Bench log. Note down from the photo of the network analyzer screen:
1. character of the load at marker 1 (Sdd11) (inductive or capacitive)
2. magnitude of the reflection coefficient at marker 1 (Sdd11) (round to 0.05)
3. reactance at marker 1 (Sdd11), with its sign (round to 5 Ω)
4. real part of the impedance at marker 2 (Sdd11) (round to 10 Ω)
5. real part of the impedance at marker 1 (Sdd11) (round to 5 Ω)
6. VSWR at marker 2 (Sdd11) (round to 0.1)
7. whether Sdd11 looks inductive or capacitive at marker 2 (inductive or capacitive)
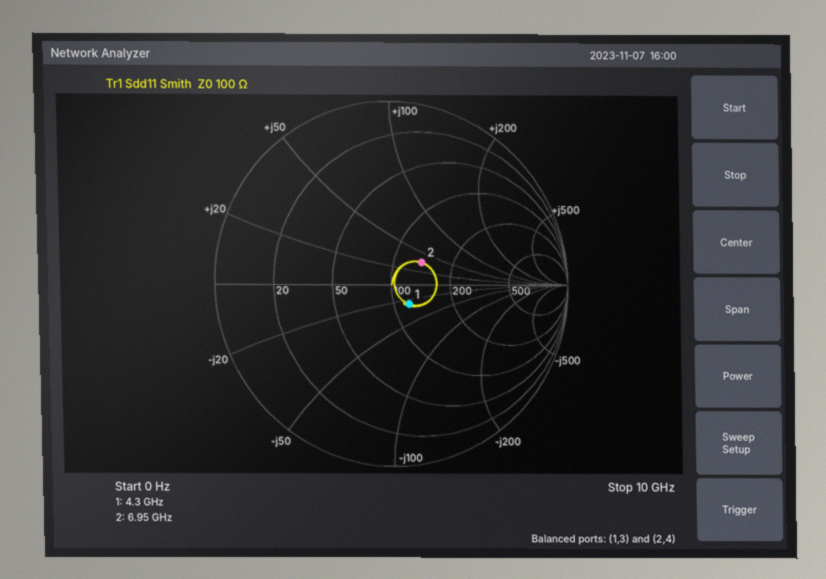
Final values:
capacitive
0.15
-25 Ω
140 Ω
120 Ω
1.5
inductive
